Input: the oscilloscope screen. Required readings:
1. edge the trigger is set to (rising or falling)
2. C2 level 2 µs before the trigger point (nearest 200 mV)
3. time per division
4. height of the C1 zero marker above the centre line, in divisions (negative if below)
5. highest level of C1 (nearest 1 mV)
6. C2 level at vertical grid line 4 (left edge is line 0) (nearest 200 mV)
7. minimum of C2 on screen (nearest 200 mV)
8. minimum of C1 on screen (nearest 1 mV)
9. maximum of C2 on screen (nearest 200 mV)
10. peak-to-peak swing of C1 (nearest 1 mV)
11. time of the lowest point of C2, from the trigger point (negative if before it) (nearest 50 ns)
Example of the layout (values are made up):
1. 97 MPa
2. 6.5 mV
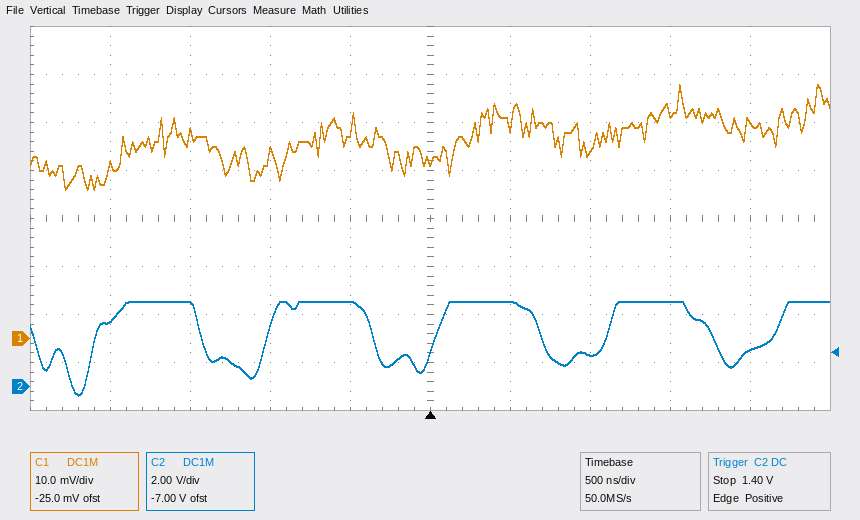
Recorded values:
1. rising
2. 2.8 V
3. 500 ns
4. -2.5 div
5. 53 mV
6. 3.6 V
7. -400 mV
8. 31 mV
9. 3.6 V
10. 22 mV
11. -2.20 µs
